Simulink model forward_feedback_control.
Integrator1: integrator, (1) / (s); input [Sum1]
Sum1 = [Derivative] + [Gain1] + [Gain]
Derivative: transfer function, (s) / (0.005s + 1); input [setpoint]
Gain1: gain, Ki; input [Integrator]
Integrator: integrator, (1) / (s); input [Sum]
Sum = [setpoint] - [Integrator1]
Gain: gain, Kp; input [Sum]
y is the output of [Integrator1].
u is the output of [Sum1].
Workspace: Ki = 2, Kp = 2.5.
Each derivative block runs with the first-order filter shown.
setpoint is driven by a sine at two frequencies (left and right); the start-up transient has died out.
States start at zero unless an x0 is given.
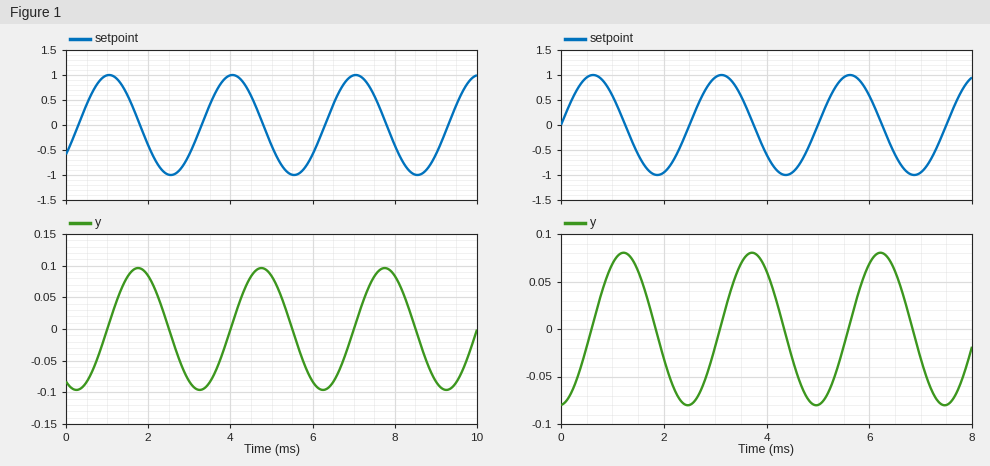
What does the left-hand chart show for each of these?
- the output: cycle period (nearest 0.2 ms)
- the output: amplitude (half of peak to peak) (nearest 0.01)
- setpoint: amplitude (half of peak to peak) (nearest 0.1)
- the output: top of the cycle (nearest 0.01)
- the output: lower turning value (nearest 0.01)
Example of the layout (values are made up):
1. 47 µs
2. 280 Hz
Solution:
1. 3.0 ms
2. 0.10
3. 1.0
4. 0.10
5. -0.10
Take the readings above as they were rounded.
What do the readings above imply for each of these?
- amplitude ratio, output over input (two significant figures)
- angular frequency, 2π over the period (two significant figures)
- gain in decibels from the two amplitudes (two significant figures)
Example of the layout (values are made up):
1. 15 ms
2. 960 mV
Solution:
1. 0.10
2. 2.1 rad/ms
3. -20 dB
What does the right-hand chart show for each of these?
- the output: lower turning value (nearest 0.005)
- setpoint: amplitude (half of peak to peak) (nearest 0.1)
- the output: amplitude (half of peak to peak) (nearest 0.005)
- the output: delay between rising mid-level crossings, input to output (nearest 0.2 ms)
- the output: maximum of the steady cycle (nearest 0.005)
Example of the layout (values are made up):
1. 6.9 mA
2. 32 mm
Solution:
1. -0.080
2. 1.0
3. 0.080
4. 0.6 ms
5. 0.080
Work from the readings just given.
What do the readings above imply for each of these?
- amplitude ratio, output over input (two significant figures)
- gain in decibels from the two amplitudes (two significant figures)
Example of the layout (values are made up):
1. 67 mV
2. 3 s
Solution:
1. 0.080
2. -22 dB
